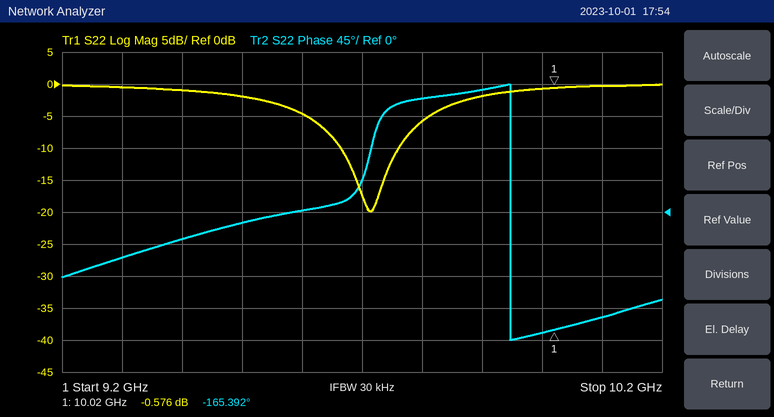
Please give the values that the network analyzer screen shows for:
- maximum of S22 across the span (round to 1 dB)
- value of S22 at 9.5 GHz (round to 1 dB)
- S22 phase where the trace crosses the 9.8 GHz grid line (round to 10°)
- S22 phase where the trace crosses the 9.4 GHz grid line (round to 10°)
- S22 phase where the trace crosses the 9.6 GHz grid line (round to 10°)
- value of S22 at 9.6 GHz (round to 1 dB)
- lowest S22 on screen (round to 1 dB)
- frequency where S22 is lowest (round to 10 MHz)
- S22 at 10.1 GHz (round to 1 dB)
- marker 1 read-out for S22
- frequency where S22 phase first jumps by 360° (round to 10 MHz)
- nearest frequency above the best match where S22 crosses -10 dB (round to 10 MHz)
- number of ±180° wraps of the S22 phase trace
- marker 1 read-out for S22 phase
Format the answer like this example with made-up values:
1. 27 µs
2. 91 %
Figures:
1. 0 dB
2. -2 dB
3. 160°
4. -40°
5. 0°
6. -5 dB
7. -20 dB
8. 9.71 GHz
9. 0 dB
10. -0.576 dB
11. 9.95 GHz
12. 9.76 GHz
13. 1
14. -165.392°
